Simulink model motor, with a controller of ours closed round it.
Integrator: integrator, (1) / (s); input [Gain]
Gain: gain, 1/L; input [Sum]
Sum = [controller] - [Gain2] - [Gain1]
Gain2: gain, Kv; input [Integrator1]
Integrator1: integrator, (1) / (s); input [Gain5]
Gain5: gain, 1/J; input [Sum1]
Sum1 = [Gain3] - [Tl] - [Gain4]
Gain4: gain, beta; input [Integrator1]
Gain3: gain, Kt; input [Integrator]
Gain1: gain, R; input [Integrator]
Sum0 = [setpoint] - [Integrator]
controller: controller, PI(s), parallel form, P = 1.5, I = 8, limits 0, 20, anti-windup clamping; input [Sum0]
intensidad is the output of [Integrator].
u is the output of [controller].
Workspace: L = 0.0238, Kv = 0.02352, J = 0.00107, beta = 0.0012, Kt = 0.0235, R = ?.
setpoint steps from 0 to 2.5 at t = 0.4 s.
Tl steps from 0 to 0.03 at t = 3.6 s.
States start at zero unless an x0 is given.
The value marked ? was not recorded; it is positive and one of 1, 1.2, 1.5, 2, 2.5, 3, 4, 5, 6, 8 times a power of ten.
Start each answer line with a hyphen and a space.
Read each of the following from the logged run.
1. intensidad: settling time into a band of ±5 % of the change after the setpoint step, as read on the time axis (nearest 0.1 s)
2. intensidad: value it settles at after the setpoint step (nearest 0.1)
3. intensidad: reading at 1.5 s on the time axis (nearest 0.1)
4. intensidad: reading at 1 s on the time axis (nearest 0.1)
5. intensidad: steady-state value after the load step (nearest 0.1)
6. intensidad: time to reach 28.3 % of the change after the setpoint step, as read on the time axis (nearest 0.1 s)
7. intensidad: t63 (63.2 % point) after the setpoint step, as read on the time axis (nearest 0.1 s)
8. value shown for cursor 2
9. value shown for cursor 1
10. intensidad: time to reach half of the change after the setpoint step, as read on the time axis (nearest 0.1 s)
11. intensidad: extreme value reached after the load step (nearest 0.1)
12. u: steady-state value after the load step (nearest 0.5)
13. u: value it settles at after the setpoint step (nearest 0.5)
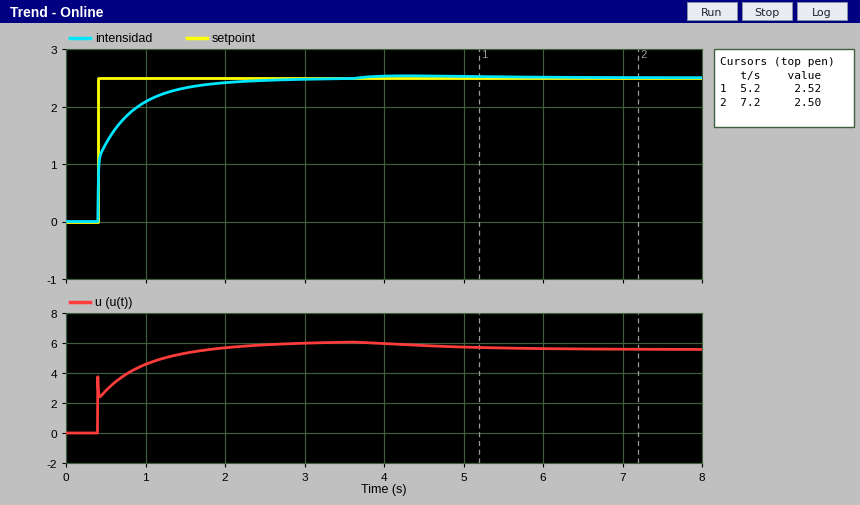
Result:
- 1.7 s
- 2.5
- 2.3
- 2.1
- 2.5
- 0.4 s
- 0.6 s
- 2.50
- 2.52
- 0.5 s
- 2.5
- 5.5
- 6.0
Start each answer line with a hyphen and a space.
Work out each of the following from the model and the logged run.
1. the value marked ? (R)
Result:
- 2
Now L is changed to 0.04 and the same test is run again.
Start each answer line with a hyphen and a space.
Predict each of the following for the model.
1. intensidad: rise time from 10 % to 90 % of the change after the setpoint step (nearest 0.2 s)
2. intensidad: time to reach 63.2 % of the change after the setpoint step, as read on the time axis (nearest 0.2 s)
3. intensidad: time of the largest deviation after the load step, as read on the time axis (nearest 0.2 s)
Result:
- 0.8 s
- 0.6 s
- 4.2 s
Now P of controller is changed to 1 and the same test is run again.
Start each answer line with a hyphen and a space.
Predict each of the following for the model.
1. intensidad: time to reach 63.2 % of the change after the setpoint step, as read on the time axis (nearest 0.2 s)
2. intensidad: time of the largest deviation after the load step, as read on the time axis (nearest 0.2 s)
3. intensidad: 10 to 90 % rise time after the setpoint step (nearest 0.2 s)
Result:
- 0.6 s
- 4.2 s
- 0.8 s
